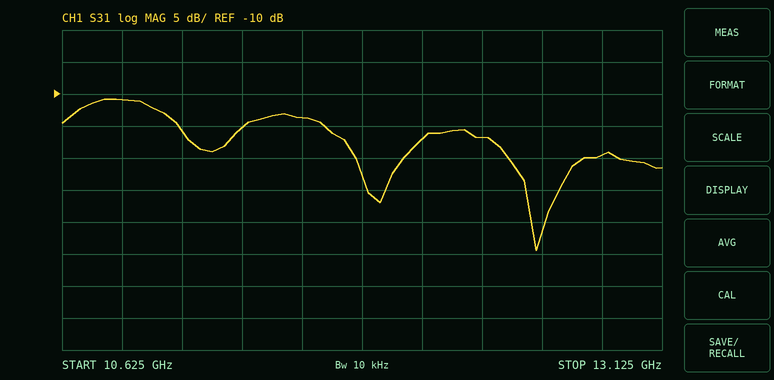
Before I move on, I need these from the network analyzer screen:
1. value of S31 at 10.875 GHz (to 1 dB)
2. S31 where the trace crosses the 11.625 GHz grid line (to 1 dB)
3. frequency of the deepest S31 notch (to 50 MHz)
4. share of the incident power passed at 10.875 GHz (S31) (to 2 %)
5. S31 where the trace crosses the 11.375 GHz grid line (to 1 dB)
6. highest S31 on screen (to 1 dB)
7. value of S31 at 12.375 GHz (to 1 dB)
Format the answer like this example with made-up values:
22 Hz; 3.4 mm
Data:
-11 dB; -14 dB; 12.60 GHz; 8 %; -15 dB; -11 dB; -17 dB
